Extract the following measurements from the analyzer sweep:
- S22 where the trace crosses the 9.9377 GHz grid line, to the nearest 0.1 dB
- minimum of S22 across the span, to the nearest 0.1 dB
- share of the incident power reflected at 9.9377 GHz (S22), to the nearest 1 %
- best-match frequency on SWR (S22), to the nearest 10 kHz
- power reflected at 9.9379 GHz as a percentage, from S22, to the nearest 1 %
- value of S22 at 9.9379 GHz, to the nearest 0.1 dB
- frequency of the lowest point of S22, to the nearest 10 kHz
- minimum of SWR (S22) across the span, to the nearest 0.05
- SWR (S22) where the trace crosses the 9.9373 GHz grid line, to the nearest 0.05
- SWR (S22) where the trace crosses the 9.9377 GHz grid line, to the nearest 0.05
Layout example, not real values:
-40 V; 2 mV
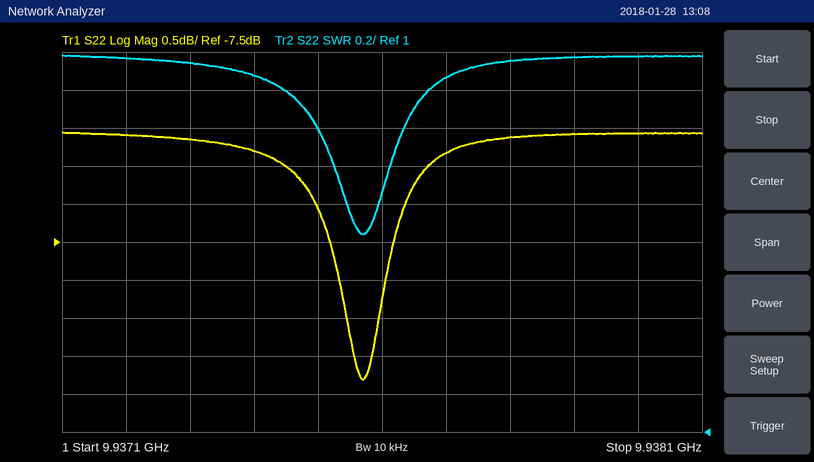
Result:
-6.3 dB; -9.3 dB; 23 %; 9.93757 GHz; 25 %; -6.1 dB; 9.93757 GHz; 2.05; 2.95; 2.85
